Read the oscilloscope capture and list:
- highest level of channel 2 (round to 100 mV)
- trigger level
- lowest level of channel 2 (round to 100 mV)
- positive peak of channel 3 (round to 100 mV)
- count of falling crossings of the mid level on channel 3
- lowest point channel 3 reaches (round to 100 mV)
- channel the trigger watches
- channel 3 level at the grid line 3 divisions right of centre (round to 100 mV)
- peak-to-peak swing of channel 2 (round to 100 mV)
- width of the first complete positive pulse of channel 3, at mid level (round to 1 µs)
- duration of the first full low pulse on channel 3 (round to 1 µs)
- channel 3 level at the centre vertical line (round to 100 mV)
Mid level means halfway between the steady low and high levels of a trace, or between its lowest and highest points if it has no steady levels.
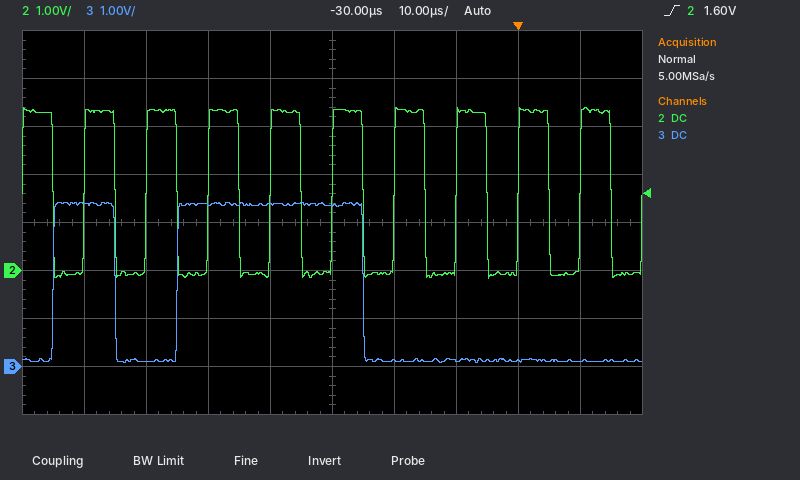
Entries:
3.4 V
1.60 V
-200 mV
3.4 V
2
100 mV
channel 2
100 mV
3.6 V
10 µs
10 µs
3.4 V
